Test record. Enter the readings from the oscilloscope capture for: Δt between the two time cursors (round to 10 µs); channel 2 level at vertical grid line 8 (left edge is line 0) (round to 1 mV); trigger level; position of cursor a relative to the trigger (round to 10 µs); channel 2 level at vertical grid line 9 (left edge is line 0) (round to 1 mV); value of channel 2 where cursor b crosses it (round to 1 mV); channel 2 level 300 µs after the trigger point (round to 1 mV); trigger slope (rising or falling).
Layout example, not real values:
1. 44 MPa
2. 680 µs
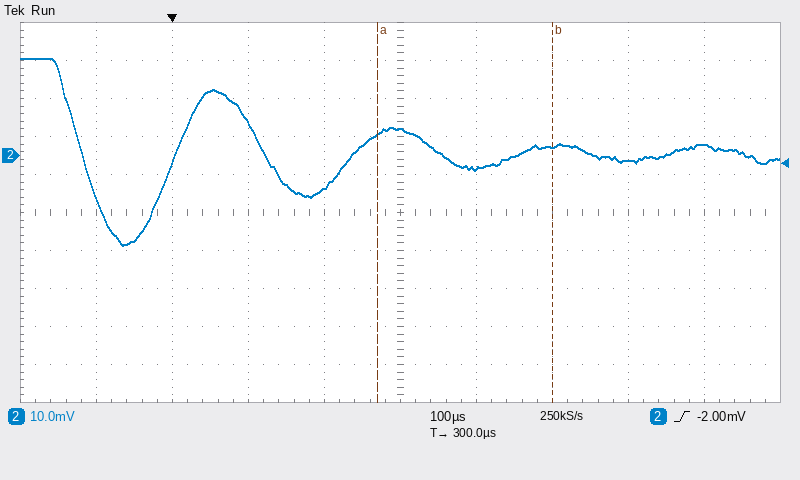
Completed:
1. 230 µs
2. -1 mV
3. -2.00 mV
4. +270 µs
5. 3 mV
6. 2 mV
7. 7 mV
8. rising
